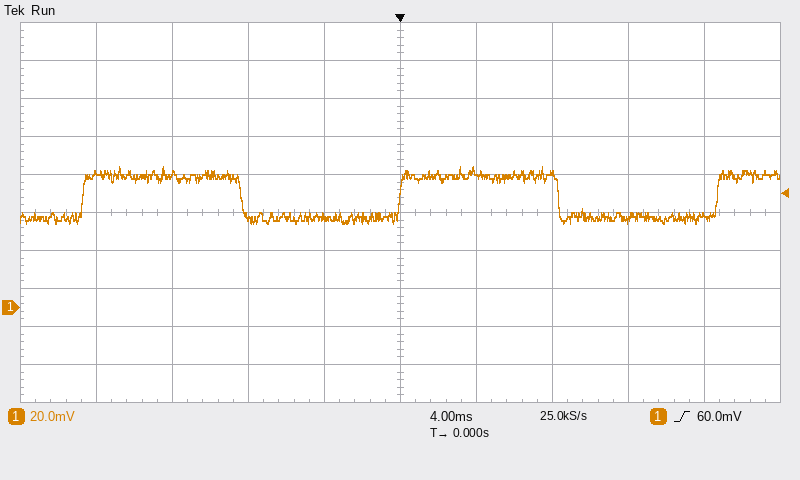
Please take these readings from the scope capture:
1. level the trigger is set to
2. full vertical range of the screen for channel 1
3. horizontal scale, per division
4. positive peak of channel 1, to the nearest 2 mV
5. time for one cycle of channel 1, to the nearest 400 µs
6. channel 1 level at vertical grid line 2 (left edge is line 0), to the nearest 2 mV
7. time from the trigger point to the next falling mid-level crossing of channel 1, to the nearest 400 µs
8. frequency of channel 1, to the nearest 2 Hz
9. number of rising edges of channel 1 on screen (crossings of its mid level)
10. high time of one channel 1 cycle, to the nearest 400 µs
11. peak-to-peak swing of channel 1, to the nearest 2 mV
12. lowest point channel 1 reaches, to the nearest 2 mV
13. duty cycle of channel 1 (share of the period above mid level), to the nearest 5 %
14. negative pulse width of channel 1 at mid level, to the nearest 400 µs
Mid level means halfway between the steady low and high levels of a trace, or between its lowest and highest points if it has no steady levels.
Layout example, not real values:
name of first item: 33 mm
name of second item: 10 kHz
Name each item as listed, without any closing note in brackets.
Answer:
level the trigger is set to: 60.0 mV
full vertical range of the screen for channel 1: 200 mV
horizontal scale, per division: 4 ms
positive peak of channel 1, to the nearest 2 mV: 74 mV
time for one cycle of channel 1, to the nearest 400 µs: 16.8 ms
channel 1 level at vertical grid line 2 (left edge is line 0), to the nearest 2 mV: 70 mV
time from the trigger point to the next falling mid-level crossing of channel 1, to the nearest 400 µs: 8.4 ms
frequency of channel 1, to the nearest 2 Hz: 60 Hz
number of rising edges of channel 1 on screen: 3
high time of one channel 1 cycle, to the nearest 400 µs: 8.4 ms
peak-to-peak swing of channel 1, to the nearest 2 mV: 30 mV
lowest point channel 1 reaches, to the nearest 2 mV: 44 mV
duty cycle of channel 1 (share of the period above mid level), to the nearest 5 %: 50 %
negative pulse width of channel 1 at mid level, to the nearest 400 µs: 8.4 ms
